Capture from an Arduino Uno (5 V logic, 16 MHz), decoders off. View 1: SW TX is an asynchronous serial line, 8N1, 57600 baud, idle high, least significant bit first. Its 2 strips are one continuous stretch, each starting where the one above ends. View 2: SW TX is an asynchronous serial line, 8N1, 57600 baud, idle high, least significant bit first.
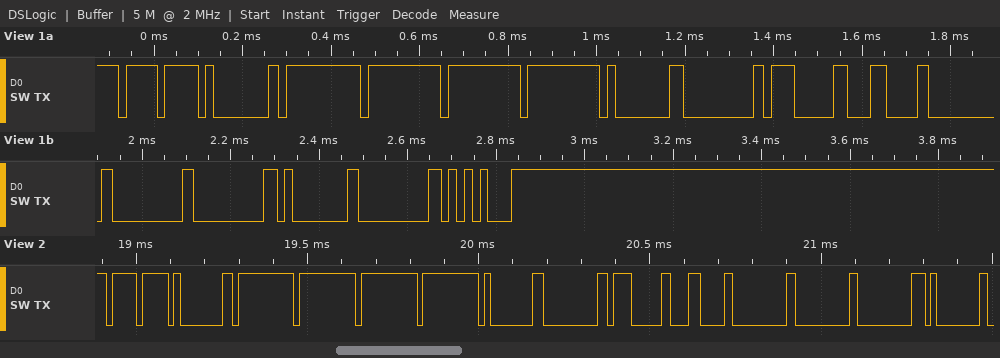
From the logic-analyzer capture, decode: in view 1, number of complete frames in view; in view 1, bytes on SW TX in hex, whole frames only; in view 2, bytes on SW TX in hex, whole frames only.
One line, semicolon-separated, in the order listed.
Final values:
16; 0xEF 0x01 0xFF 0xFF 0xFF 0xFF 0x01 0x00 0x07 0x0C 0x00 0x00 0x00 0x01 0x00 0x15; EF 01 FF FF FF FF 01 00 07 0C 00 00 00 01
